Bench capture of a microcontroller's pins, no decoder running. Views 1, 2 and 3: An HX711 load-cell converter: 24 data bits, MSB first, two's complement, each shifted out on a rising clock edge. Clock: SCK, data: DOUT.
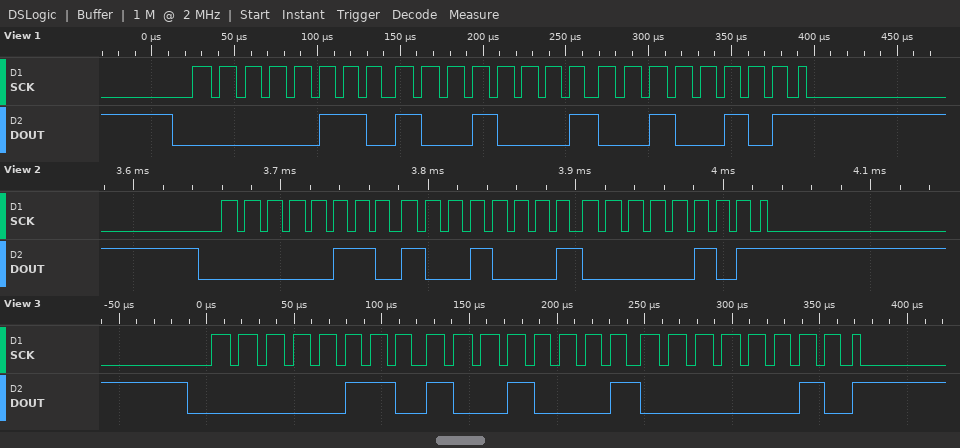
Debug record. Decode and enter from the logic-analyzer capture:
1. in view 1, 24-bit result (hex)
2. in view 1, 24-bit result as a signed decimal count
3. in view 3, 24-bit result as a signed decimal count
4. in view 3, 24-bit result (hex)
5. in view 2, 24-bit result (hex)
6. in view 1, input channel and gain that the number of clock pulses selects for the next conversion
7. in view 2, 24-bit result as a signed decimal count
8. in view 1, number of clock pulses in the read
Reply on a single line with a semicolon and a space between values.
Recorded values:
0x069125; 430373; 430338; 0x069102; 0x069105; channel A, gain 128; 430341; 25
